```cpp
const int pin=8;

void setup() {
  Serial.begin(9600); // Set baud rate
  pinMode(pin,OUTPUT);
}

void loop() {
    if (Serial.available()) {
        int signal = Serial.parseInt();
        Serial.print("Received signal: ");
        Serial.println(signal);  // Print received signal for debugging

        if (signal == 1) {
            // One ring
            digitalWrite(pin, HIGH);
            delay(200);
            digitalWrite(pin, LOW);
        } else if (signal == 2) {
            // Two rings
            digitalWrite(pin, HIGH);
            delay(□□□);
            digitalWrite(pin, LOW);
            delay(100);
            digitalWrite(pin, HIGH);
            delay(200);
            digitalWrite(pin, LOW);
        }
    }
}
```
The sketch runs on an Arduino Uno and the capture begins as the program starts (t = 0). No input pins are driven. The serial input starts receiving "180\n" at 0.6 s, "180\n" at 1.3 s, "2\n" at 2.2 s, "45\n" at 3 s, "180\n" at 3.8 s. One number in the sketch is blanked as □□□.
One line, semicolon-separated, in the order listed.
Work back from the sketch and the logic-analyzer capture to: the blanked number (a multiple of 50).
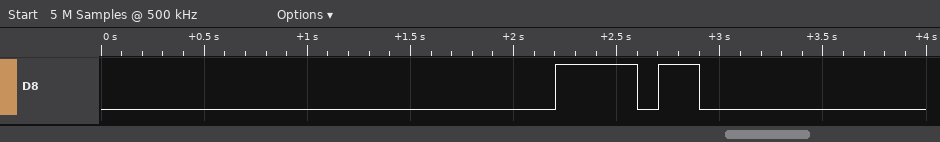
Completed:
400
